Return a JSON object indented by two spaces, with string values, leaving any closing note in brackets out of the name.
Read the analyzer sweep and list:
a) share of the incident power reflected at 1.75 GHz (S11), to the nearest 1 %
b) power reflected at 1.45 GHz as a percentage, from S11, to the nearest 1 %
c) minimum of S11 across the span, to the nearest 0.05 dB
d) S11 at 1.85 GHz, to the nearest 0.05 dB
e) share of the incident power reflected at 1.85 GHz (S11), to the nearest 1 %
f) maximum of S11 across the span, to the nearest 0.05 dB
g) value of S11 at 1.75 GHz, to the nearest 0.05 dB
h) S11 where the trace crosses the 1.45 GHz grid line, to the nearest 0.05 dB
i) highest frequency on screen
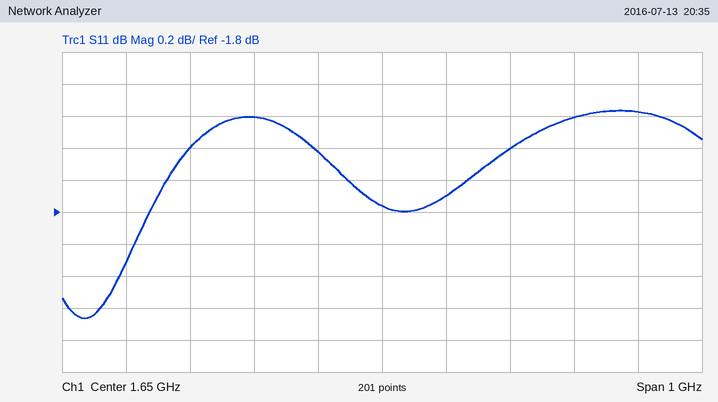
{
  "share of the incident power reflected at 1.75 GHz (S11), to the nearest 1 %": "68 %",
  "power reflected at 1.45 GHz as a percentage, from S11, to the nearest 1 %": "76 %",
  "minimum of S11 across the span, to the nearest 0.05 dB": "-2.45 dB",
  "S11 at 1.85 GHz, to the nearest 0.05 dB": "-1.40 dB",
  "share of the incident power reflected at 1.85 GHz (S11), to the nearest 1 %": "72 %",
  "maximum of S11 across the span, to the nearest 0.05 dB": "-1.15 dB",
  "value of S11 at 1.75 GHz, to the nearest 0.05 dB": "-1.70 dB",
  "S11 where the trace crosses the 1.45 GHz grid line, to the nearest 0.05 dB": "-1.20 dB",
  "highest frequency on screen": "2.15 GHz"
}
